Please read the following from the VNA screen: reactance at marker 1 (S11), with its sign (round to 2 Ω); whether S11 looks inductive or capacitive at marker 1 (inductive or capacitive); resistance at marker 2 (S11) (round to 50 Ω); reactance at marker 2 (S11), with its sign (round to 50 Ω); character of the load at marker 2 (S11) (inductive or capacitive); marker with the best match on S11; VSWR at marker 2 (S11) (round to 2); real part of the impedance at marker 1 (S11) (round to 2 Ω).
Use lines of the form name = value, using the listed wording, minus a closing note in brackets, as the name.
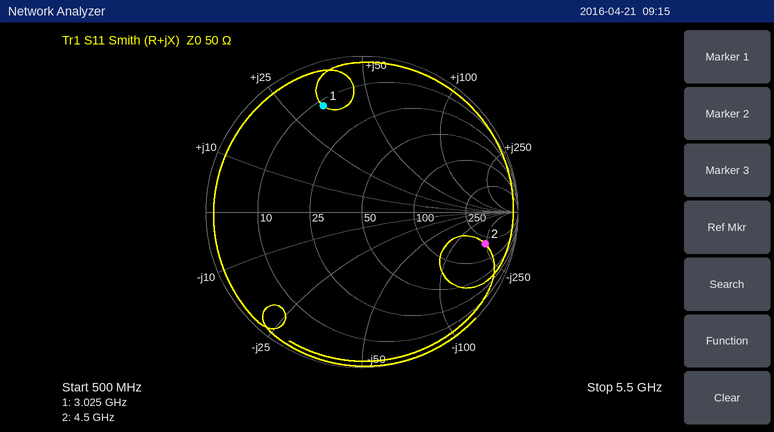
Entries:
reactance at marker 1 (S11), with its sign = +34 Ω
whether S11 looks inductive or capacitive at marker 1 = inductive
resistance at marker 2 (S11) = 200 Ω
reactance at marker 2 (S11), with its sign = -250 Ω
character of the load at marker 2 (S11) = capacitive
marker with the best match on S11 = marker 1
VSWR at marker 2 (S11) = 10
real part of the impedance at marker 1 (S11) = 12 Ω
